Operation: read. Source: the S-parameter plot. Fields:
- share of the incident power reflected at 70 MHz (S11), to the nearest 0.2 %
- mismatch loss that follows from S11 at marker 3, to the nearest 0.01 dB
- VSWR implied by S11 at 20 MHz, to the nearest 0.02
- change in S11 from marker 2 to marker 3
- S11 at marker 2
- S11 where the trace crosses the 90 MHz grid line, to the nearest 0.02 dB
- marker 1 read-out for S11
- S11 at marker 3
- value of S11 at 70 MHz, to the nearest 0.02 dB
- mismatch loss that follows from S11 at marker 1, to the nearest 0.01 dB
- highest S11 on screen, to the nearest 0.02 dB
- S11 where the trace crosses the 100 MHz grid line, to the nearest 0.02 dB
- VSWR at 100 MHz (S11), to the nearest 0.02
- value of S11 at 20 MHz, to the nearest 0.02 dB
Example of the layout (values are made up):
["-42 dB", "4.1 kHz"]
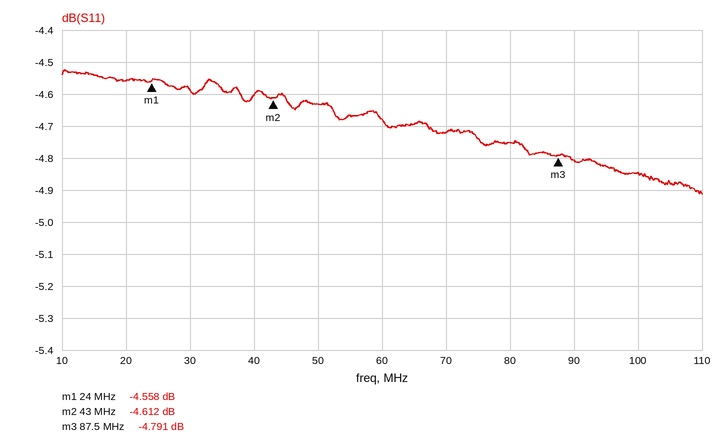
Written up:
["33.8 %", "1.75 dB", "3.90", "-0.179 dB", "-4.612 dB", "-4.80 dB", "-4.558 dB", "-4.791 dB", "-4.72 dB", "1.87 dB", "-4.52 dB", "-4.84 dB", "3.68", "-4.56 dB"]
